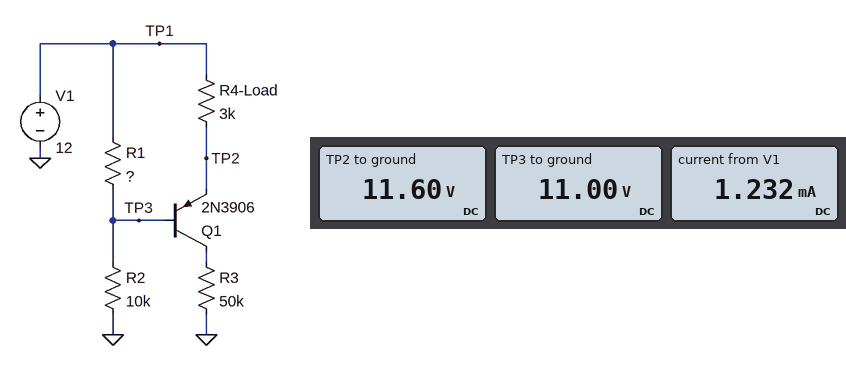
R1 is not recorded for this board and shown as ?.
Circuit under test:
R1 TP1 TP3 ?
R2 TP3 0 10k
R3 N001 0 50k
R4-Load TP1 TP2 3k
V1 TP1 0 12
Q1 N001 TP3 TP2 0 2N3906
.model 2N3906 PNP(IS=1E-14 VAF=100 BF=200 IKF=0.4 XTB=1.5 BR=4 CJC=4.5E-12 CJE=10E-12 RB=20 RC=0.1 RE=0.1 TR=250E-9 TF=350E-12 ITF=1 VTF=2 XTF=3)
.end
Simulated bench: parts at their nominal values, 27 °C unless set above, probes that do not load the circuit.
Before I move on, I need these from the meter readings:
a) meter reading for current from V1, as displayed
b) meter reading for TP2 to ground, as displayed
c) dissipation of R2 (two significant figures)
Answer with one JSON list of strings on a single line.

["1.232 mA", "11.60 V", "12 mW"]
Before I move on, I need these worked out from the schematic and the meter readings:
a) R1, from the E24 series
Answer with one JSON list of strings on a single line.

["910 Ω"]
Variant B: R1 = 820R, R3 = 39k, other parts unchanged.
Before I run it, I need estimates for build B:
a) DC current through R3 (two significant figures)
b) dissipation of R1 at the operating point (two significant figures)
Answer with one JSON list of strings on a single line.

["100 µA", "1.0 mW"]
